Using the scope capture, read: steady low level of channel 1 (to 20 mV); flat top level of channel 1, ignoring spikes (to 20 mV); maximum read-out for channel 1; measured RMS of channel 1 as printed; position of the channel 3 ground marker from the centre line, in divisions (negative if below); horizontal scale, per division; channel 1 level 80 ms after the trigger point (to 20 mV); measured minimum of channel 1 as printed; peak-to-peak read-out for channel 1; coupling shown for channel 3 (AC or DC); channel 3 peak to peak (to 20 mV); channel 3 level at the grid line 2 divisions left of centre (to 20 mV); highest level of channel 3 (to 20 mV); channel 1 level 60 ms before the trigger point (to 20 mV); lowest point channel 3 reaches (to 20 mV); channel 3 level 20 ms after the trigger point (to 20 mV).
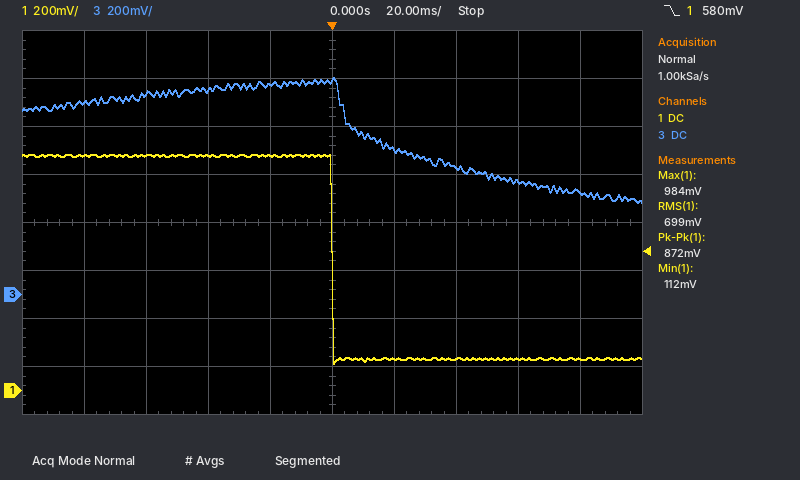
140 mV
980 mV
984 mV
699 mV
-1.5 div
20 ms
140 mV
112 mV
872 mV
DC
520 mV
860 mV
900 mV
980 mV
380 mV
600 mV
